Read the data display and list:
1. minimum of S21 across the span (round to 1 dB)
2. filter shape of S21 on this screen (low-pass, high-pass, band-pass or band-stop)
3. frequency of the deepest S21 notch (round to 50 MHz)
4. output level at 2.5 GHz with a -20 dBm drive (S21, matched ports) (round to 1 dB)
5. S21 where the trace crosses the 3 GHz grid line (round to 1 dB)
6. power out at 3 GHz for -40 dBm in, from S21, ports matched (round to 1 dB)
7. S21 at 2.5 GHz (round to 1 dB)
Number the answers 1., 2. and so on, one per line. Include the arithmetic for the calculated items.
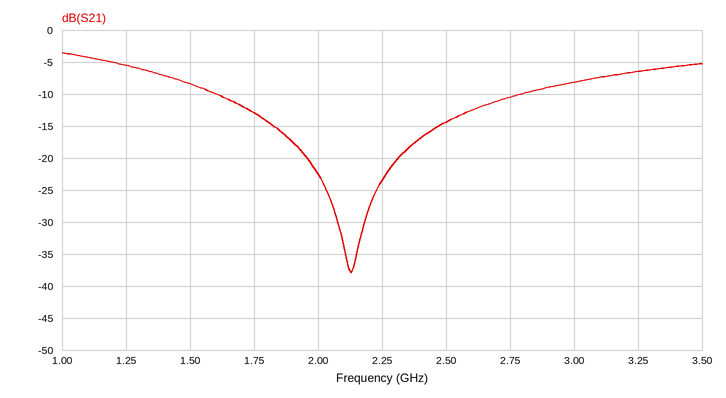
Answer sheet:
1. -38 dB
2. band-stop
3. 2.15 GHz
4. -20 dBm + (-14 dB) = -34 dBm
5. -8 dB
6. -40 dBm + (-8 dB) = -48 dBm
7. -14 dB
